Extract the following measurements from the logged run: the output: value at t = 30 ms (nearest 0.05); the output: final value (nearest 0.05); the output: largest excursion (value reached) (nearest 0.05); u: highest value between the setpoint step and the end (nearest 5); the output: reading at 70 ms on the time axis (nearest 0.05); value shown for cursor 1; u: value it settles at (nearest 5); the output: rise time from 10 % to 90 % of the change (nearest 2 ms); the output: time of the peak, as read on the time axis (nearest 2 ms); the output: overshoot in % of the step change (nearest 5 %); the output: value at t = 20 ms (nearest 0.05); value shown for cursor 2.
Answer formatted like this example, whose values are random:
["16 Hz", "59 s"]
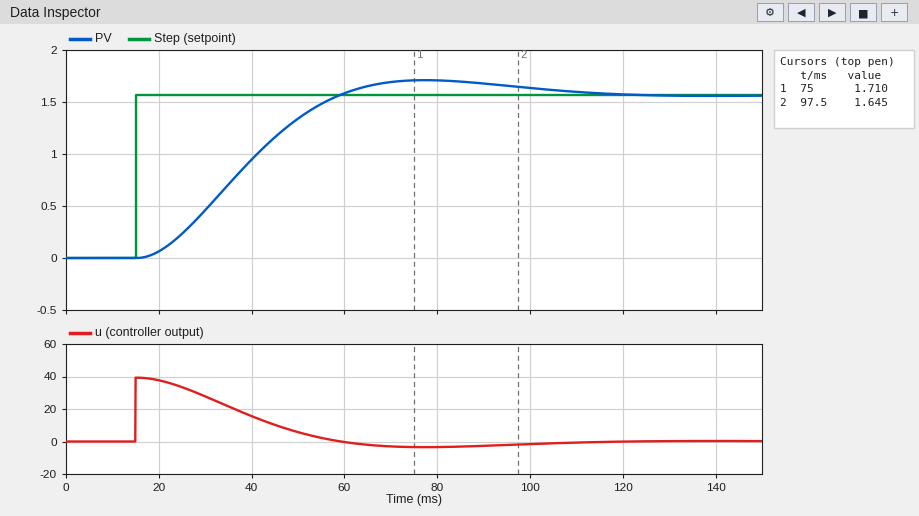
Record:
["0.45", "1.55", "1.70", "40", "1.70", "1.710", "0", "30 ms", "78 ms", "10 %", "0.05", "1.645"]
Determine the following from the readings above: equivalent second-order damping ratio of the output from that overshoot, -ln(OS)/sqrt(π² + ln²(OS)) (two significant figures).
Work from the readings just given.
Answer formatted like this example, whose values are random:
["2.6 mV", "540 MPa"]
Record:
["0.59"]
